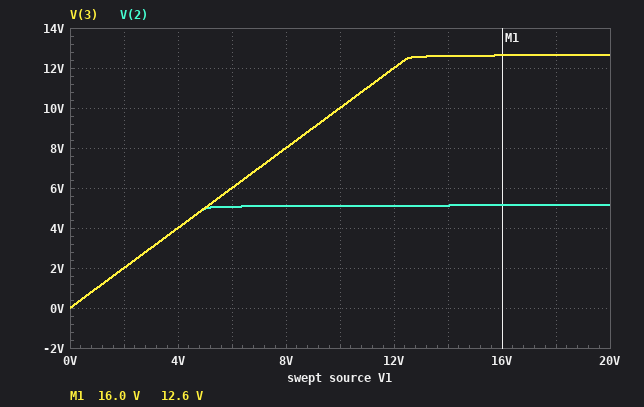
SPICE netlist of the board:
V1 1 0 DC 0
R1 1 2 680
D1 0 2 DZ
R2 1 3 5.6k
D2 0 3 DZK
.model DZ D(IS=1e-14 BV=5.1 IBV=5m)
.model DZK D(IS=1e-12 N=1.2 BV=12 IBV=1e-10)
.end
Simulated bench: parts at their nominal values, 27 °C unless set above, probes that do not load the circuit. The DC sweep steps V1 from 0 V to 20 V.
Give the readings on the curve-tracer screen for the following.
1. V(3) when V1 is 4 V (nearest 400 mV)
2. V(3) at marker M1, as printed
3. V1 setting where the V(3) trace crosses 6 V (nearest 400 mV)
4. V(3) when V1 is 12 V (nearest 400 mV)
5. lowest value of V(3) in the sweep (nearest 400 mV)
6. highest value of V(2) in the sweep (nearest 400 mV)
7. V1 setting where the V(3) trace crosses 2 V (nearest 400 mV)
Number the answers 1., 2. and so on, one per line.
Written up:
1. 4.0 V
2. 12.6 V
3. 6.0 V
4. 12.0 V
5. 0 V
6. 5.2 V
7. 2.0 V
